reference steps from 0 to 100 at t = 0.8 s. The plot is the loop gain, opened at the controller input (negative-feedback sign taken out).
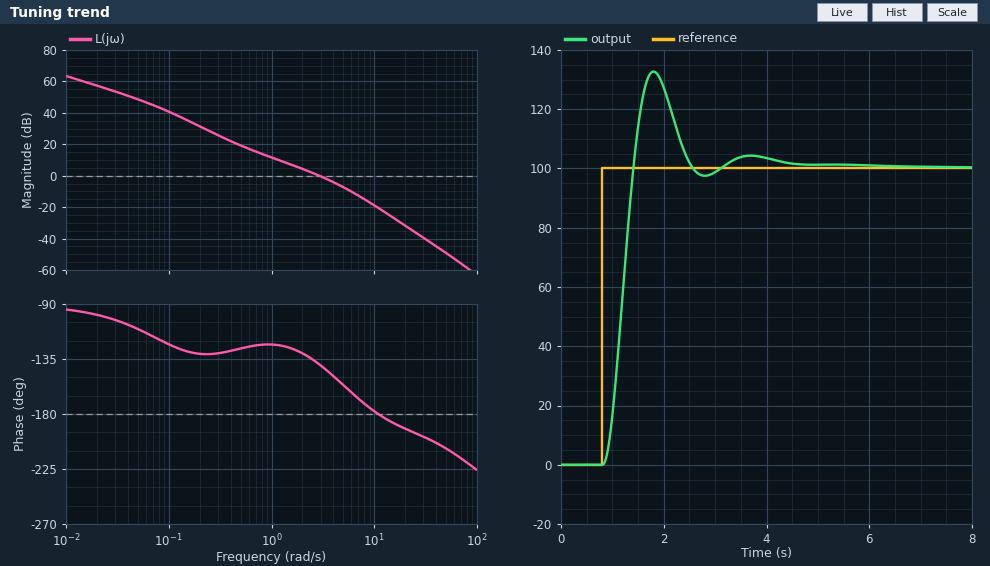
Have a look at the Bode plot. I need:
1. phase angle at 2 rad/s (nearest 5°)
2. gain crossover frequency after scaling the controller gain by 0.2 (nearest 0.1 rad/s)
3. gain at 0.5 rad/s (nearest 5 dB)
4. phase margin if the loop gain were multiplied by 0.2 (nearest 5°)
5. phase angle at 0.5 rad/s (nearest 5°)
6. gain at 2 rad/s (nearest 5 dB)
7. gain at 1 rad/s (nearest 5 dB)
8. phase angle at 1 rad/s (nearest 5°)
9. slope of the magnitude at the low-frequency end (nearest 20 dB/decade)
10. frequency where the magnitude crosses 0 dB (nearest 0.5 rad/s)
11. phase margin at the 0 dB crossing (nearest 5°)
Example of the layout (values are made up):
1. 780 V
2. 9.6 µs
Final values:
1. -130°
2. 0.8 rad/s
3. 20 dB
4. 55°
5. -125°
6. 5 dB
7. 10 dB
8. -125°
9. -20 dB/decade
10. 3.0 rad/s
11. 40°
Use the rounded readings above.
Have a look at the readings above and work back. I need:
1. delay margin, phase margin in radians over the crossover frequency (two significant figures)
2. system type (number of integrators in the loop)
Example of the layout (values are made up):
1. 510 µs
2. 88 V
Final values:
1. 0.23 s
2. 1
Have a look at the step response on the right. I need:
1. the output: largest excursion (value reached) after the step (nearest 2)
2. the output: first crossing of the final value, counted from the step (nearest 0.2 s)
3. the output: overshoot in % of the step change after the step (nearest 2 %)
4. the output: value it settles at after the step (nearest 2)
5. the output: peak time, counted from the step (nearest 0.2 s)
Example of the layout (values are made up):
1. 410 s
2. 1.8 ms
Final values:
1. 132
2. 0.6 s
3. 32 %
4. 100
5. 1.0 s
